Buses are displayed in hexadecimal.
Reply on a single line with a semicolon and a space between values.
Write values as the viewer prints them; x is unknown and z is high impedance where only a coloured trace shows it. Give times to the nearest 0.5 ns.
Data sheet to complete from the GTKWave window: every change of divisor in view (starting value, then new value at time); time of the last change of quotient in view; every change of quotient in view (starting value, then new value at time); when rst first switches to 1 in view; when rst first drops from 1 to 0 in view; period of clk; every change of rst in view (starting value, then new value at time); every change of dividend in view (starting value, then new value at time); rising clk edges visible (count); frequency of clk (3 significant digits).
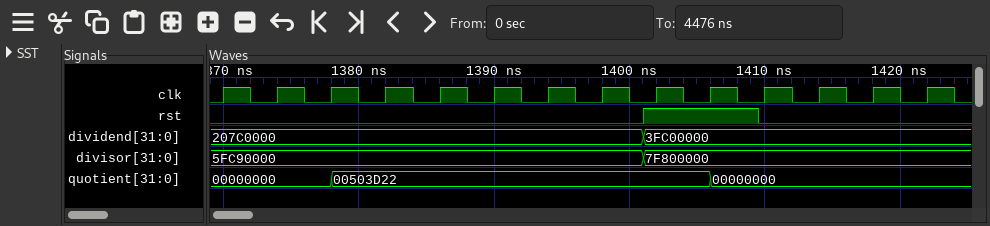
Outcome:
5FC90000, 7F800000 at 1401 ns; 1406 ns; 00000000, 00503D22 at 1378 ns, 00000000 at 1406 ns; 1401 ns; 1409.5 ns; 4 ns; 0, 1 at 1401 ns, 0 at 1409.5 ns; 207C0000, 3FC00000 at 1401 ns; 14; 250 MHz
